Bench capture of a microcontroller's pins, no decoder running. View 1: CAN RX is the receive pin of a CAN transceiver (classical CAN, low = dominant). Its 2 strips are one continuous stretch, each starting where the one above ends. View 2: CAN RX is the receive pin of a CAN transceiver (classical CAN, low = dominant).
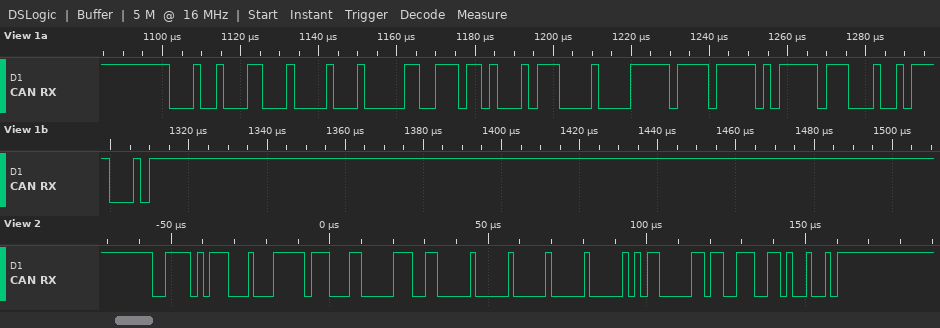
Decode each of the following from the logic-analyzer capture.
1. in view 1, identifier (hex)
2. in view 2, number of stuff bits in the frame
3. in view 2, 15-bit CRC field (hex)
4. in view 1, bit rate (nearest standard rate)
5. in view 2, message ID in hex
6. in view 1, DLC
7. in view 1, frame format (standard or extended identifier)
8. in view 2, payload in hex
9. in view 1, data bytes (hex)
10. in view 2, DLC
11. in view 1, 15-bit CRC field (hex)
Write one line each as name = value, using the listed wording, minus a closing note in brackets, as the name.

in view 1, identifier = 0x123
in view 2, number of stuff bits in the frame = 8
in view 2, 15-bit CRC field = 0x39A4
in view 1, bit rate = 500 kbit/s
in view 2, message ID in hex = 0x3D7
in view 1, DLC = 8
in view 1, frame format = standard
in view 2, payload in hex = FF 18 33 00 00 00 2C 16
in view 1, data bytes = 44 13 B4 5C 21 FF 7E FF
in view 2, DLC = 8
in view 1, 15-bit CRC field = 0x0978
